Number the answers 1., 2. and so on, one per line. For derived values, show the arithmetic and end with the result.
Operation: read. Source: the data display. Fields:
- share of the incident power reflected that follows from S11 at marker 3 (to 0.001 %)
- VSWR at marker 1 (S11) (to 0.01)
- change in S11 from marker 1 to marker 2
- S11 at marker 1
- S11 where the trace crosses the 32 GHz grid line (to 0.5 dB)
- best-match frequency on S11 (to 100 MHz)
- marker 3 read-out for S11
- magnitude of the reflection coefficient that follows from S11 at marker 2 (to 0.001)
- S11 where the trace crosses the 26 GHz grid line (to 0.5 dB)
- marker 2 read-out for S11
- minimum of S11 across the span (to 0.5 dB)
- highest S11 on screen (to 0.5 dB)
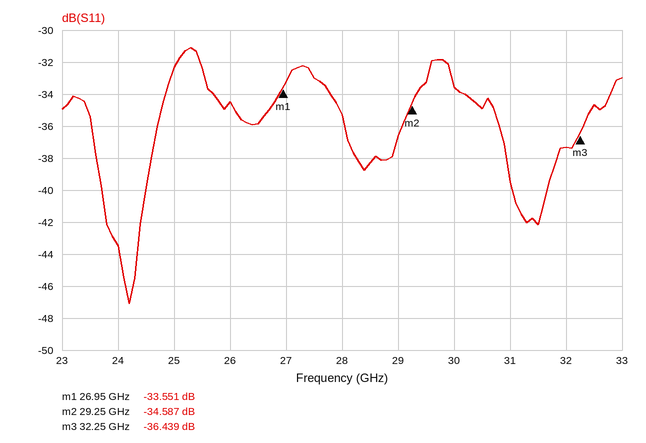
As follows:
1. 10^(-36.439/10) ≈ 0.023 %
2. (1 + 0.0210)/(1 − 0.0210) ≈ 1.04
3. -34.587 − (-33.551) = -1.036 dB
4. -33.551 dB
5. -37.5 dB
6. 24.2 GHz
7. -36.439 dB
8. 10^(-34.587/20) ≈ 0.019
9. -34.5 dB
10. -34.587 dB
11. -47.0 dB
12. -31.0 dB
